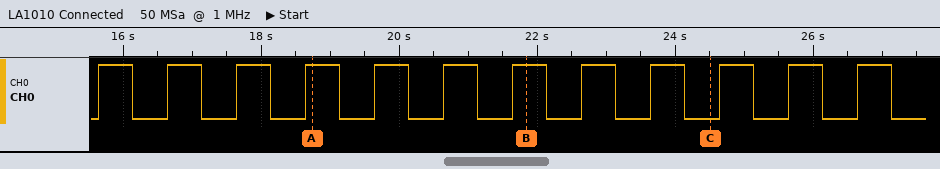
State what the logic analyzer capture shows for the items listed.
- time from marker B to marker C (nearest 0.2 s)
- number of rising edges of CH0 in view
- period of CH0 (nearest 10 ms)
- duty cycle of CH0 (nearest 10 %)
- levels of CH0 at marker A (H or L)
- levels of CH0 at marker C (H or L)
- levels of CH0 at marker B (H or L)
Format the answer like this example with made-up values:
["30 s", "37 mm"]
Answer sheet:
["2.6 s", "12", "1000 ms", "50 %", "CH0=H", "CH0=L", "CH0=H"]
